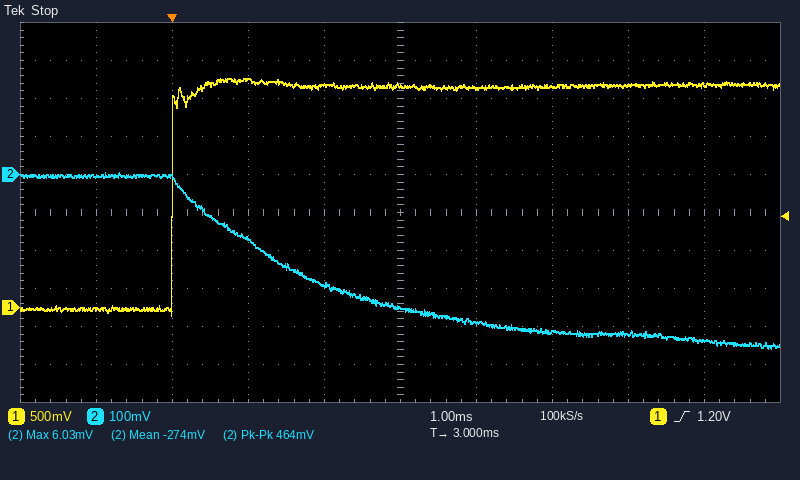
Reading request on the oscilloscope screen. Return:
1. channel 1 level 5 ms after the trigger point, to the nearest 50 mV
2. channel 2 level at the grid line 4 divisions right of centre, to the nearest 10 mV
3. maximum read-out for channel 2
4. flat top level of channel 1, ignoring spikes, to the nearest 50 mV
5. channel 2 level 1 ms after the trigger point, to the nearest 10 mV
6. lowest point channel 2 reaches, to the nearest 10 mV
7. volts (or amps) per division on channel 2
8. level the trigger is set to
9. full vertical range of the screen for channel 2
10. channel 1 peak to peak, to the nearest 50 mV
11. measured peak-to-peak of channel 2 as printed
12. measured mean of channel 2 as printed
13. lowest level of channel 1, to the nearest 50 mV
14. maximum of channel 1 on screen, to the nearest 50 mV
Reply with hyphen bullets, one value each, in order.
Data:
- 2.90 V
- -440 mV
- 6.03 mV
- 2.90 V
- -170 mV
- -460 mV
- 100 mV
- 1.20 V
- 1 V
- 3.10 V
- 464 mV
- -274 mV
- -100 mV
- 3.00 V
